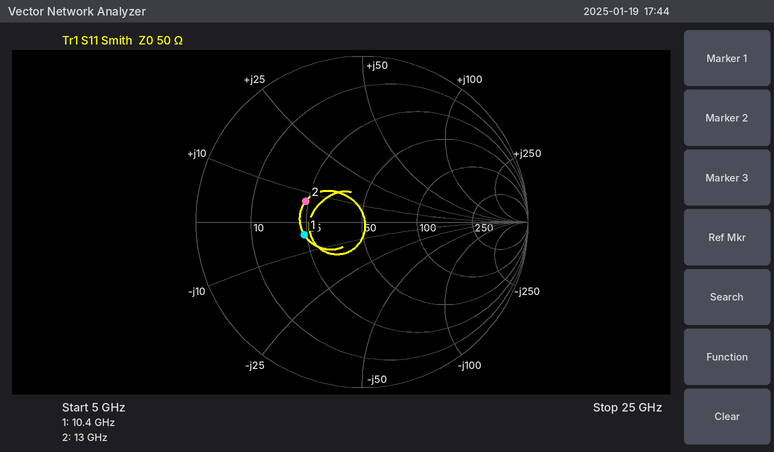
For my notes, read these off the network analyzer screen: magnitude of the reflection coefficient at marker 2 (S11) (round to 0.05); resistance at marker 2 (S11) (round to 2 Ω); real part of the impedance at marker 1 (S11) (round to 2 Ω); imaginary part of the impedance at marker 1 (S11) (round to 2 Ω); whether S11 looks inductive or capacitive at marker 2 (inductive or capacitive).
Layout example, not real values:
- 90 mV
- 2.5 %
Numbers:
- 0.35
- 24 Ω
- 24 Ω
- -4 Ω
- inductive
